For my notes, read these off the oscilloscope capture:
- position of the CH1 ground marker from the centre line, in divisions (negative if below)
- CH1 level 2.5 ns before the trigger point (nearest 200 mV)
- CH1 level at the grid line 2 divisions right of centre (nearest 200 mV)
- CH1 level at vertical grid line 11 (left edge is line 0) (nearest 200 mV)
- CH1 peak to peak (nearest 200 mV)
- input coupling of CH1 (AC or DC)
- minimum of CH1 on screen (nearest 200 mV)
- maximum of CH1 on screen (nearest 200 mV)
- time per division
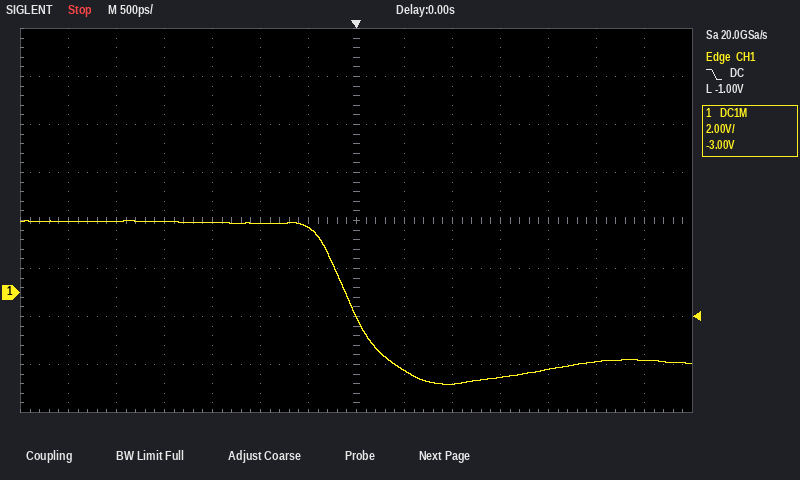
-1.5 div
3.0 V
-3.8 V
-3.2 V
6.8 V
DC
-3.8 V
3.0 V
500 ps
